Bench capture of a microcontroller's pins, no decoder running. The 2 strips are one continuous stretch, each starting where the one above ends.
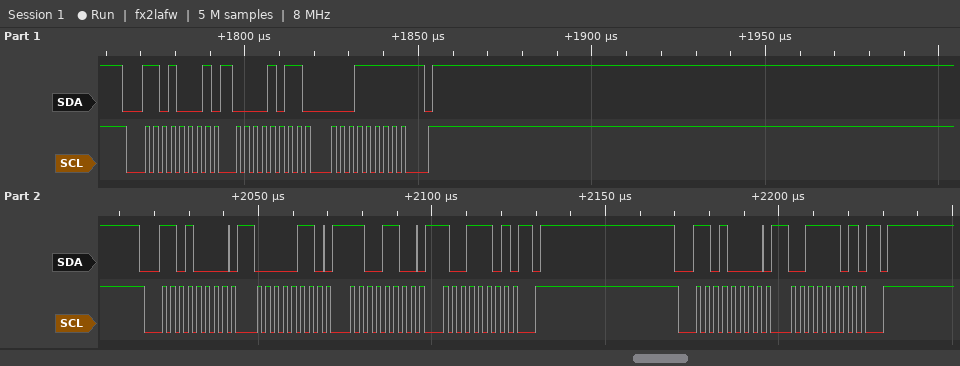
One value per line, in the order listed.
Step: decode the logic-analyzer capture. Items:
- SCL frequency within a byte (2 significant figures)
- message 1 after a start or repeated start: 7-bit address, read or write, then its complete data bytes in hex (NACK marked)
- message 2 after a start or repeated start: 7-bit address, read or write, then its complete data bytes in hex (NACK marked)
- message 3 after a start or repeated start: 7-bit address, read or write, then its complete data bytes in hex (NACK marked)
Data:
400 kHz
0x68 read: 0B 1F NACK
0x68 write: 06 CC 9D
0x68 write: 3D
